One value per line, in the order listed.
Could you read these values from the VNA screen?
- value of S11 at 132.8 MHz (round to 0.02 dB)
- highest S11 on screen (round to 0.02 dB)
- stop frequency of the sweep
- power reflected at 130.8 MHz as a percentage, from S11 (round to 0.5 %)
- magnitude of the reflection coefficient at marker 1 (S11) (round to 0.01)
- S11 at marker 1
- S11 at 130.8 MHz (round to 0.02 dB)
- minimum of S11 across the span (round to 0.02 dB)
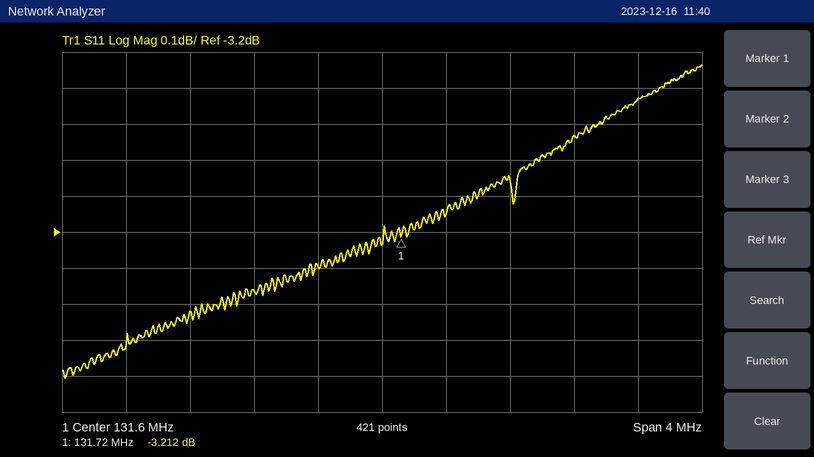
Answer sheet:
-2.94 dB
-2.74 dB
133.6 MHz
46.0 %
0.69
-3.212 dB
-3.36 dB
-3.60 dB
